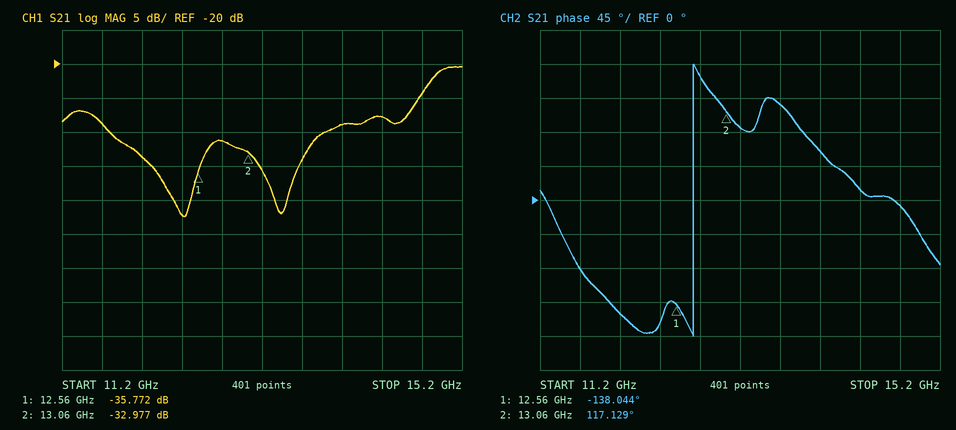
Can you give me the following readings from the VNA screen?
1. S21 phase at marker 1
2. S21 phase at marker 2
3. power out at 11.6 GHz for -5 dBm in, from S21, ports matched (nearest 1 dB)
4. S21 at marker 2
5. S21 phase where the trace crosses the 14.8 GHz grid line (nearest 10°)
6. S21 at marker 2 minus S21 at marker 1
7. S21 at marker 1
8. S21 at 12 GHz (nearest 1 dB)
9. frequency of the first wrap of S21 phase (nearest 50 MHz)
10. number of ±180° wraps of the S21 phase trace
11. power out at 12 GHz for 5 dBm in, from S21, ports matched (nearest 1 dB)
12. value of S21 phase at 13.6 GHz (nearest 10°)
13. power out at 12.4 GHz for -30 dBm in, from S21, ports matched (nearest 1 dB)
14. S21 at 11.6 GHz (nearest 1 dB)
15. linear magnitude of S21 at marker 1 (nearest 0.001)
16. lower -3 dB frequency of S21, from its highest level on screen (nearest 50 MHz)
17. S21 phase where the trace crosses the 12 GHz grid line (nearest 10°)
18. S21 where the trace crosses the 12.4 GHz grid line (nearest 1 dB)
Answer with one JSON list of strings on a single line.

["-138.044°", "117.129°", "-34 dBm", "-32.977 dB", "-10°", "2.795 dB", "-35.772 dB", "-34 dB", "12.75 GHz", "1", "-29 dBm", "130°", "-72 dBm", "-29 dB", "0.016", "14.85 GHz", "-150°", "-42 dB"]
